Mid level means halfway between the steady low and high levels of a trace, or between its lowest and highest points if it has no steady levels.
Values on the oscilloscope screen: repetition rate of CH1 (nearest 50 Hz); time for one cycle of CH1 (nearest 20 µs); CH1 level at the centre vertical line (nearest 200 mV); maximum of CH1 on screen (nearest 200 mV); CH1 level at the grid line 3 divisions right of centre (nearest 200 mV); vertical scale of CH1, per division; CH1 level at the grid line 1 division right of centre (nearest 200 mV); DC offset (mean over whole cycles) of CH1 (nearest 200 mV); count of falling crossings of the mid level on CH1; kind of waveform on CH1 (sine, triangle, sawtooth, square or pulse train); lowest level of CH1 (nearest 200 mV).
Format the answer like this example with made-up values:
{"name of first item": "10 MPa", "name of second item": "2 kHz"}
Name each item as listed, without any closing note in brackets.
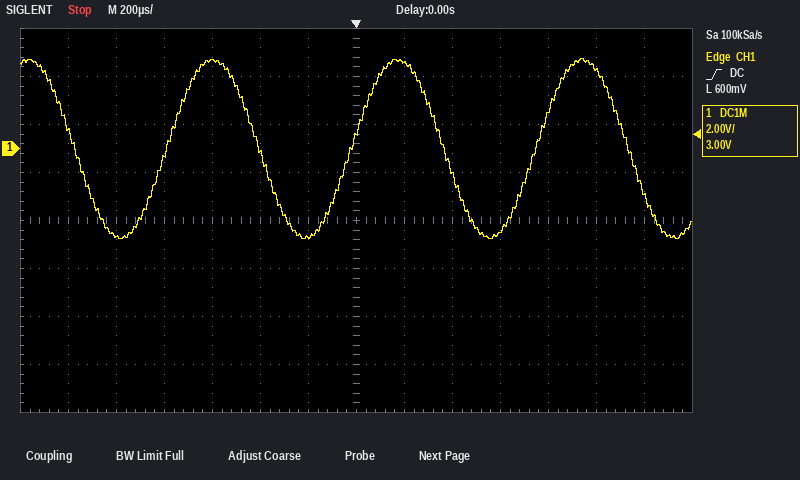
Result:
{"repetition rate of CH1": "1.30 kHz", "time for one cycle of CH1": "760 µs", "CH1 level at the centre vertical line": "600 mV", "maximum of CH1 on screen": "3.8 V", "CH1 level at the grid line 3 divisions right of centre": "-3.4 V", "vertical scale of CH1, per division": "2 V", "CH1 level at the grid line 1 division right of centre": "3.6 V", "DC offset (mean over whole cycles) of CH1": "0.0 V", "count of falling crossings of the mid level on CH1": "4", "kind of waveform on CH1": "sine", "lowest level of CH1": "-3.8 V"}
